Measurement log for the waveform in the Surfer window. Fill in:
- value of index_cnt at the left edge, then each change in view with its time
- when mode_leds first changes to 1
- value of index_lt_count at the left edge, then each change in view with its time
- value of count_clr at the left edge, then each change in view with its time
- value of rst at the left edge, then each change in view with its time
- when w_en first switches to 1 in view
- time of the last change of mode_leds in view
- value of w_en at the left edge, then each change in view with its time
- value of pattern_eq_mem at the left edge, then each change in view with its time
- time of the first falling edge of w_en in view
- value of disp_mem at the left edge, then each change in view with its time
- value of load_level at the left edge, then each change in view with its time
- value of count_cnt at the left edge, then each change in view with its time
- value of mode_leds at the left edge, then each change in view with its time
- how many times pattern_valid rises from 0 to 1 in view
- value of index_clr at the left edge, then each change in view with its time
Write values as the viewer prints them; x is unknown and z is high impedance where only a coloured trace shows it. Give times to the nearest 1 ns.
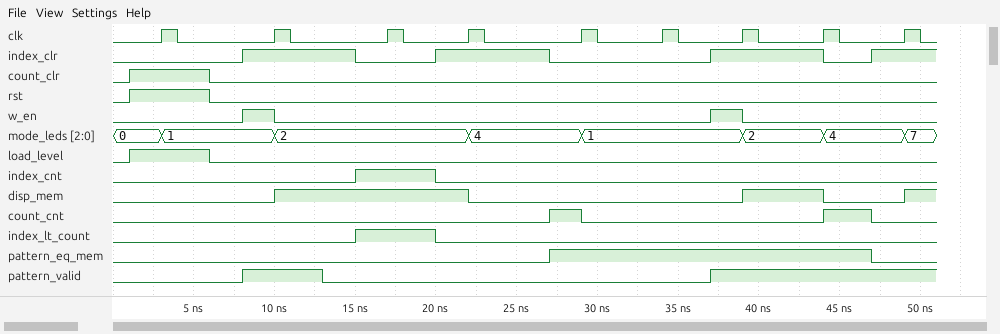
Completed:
0, 1 at 15 ns, 0 at 20 ns
3 ns
0, 1 at 15 ns, 0 at 20 ns
0, 1 at 1 ns, 0 at 6 ns
0, 1 at 1 ns, 0 at 6 ns
8 ns
49 ns
0, 1 at 8 ns, 0 at 10 ns, 1 at 37 ns, 0 at 39 ns
0, 1 at 27 ns, 0 at 47 ns
10 ns
0, 1 at 10 ns, 0 at 22 ns, 1 at 39 ns, 0 at 44 ns, 1 at 49 ns
0, 1 at 1 ns, 0 at 6 ns
0, 1 at 27 ns, 0 at 29 ns, 1 at 44 ns, 0 at 47 ns
0, 1 at 3 ns, 2 at 10 ns, 4 at 22 ns, 1 at 29 ns, 2 at 39 ns, 4 at 44 ns, 7 at 49 ns
2
0, 1 at 8 ns, 0 at 15 ns, 1 at 20 ns, 0 at 27 ns, 1 at 37 ns, 0 at 44 ns, 1 at 47 ns
